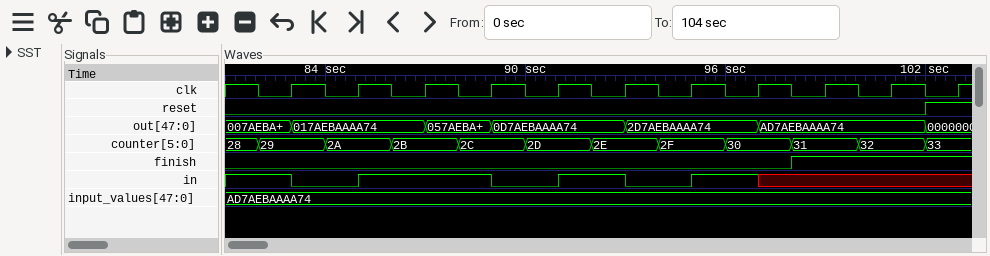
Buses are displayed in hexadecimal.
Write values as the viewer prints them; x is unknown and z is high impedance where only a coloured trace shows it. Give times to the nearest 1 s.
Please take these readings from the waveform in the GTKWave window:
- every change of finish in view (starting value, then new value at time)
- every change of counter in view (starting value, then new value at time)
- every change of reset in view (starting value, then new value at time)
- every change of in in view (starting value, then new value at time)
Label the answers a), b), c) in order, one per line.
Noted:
a) 0, 1 at 98 s
b) 28, 29 at 82 s, 2A at 84 s, 2B at 86 s, 2C at 88 s, 2D at 90 s, 2E at 92 s, 2F at 94 s, 30 at 96 s, 31 at 98 s, 32 at 100 s, 33 at 102 s
c) 0, 1 at 102 s
d) 1, 0 at 83 s, 1 at 85 s, 0 at 89 s, 1 at 91 s, 0 at 93 s, 1 at 95 s, x at 97 s
